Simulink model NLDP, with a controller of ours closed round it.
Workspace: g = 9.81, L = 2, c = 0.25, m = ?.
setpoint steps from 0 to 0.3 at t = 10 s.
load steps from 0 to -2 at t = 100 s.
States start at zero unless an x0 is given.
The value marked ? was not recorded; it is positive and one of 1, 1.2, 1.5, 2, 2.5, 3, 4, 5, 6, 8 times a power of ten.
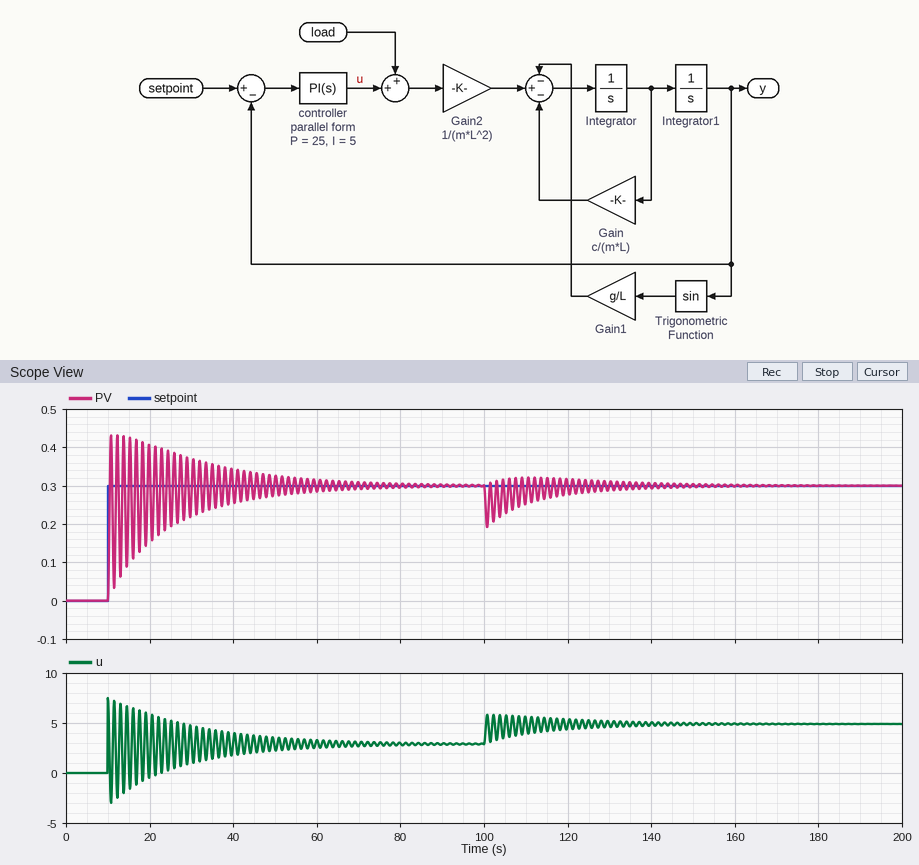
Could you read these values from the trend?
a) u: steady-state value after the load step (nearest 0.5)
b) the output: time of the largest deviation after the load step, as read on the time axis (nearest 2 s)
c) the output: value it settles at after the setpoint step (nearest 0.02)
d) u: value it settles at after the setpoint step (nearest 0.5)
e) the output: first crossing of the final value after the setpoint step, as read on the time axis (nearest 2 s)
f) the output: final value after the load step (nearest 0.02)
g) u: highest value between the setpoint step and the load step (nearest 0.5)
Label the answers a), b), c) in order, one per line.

a) 5.0
b) 100 s
c) 0.30
d) 3.0
e) 10 s
f) 0.30
g) 7.5
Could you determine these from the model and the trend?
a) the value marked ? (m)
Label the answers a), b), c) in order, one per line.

a) 0.5
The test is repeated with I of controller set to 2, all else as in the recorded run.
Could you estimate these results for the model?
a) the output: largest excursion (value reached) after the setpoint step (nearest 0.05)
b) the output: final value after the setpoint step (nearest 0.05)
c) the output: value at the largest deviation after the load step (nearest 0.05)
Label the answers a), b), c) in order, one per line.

a) 0.40
b) 0.30
c) 0.20
